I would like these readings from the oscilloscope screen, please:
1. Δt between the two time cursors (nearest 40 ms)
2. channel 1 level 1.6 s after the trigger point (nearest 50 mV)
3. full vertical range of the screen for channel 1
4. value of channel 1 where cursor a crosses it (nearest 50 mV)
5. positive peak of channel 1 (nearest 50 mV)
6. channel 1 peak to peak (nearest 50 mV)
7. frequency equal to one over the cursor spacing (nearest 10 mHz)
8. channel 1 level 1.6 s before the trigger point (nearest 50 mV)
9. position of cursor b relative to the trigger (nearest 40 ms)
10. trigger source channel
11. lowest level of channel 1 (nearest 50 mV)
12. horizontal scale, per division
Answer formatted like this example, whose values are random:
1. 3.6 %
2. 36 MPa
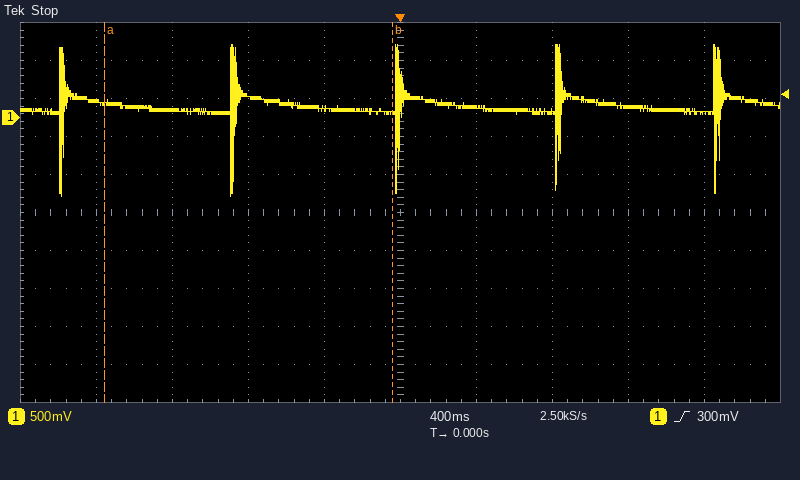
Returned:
1. 1.52 s
2. 50 mV
3. 5 V
4. 200 mV
5. 950 mV
6. 2.00 V
7. 660 mHz
8. 200 mV
9. -40 ms
10. channel 1
11. -1.05 V
12. 400 ms
